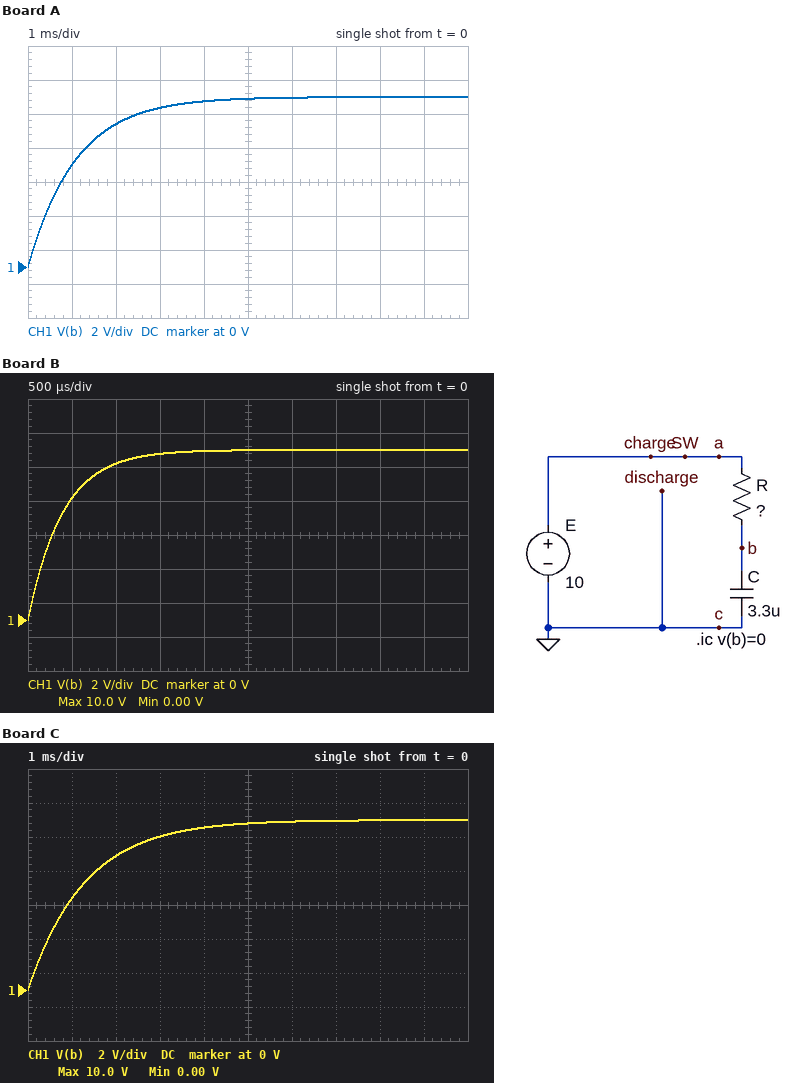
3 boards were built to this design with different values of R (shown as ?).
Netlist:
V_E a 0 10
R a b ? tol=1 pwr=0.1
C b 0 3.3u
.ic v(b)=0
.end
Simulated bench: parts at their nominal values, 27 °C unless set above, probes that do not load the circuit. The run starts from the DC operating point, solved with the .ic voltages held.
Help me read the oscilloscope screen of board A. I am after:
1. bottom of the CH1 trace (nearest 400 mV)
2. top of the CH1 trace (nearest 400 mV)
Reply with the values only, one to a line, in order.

0 V
10.0 V
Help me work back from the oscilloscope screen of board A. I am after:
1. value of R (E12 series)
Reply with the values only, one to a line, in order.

330 Ω
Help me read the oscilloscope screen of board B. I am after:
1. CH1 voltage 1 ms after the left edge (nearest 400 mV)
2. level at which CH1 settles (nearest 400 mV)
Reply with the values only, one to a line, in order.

9.2 V
10.0 V
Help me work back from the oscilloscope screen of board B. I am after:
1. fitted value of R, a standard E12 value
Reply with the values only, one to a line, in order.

120 Ω
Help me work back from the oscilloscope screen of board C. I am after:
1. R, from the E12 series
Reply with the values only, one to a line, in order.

390 Ω
